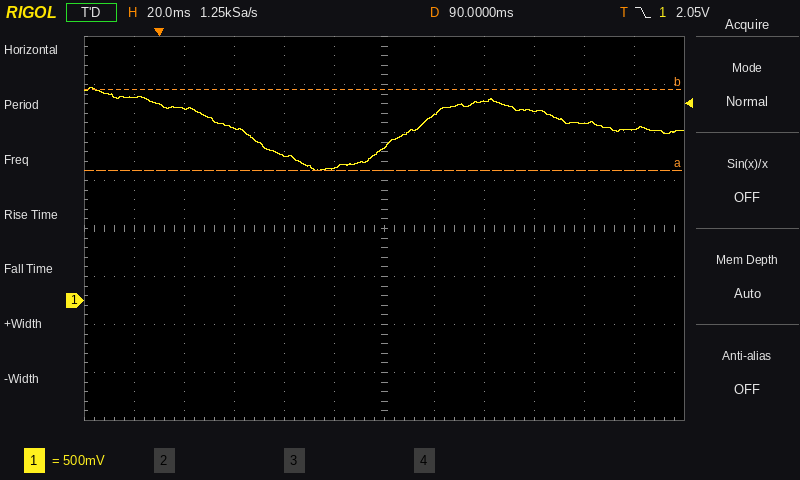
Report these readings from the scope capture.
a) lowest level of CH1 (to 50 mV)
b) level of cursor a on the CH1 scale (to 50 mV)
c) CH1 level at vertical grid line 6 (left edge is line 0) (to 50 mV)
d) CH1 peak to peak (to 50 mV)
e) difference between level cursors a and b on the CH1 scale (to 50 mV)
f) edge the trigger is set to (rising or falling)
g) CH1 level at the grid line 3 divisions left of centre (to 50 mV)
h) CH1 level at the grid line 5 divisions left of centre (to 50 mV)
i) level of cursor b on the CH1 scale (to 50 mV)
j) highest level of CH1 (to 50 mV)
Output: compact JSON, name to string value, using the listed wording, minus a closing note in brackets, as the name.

{"lowest level of CH1": "1.35 V", "level of cursor a on the CH1 scale": "1.35 V", "CH1 level at vertical grid line 6 (left edge is line 0)": "1.60 V", "CH1 peak to peak": "850 mV", "difference between level cursors a and b on the CH1 scale": "850 mV", "edge the trigger is set to": "falling", "CH1 level at the grid line 3 divisions left of centre": "1.80 V", "CH1 level at the grid line 5 divisions left of centre": "2.10 V", "level of cursor b on the CH1 scale": "2.20 V", "highest level of CH1": "2.20 V"}
